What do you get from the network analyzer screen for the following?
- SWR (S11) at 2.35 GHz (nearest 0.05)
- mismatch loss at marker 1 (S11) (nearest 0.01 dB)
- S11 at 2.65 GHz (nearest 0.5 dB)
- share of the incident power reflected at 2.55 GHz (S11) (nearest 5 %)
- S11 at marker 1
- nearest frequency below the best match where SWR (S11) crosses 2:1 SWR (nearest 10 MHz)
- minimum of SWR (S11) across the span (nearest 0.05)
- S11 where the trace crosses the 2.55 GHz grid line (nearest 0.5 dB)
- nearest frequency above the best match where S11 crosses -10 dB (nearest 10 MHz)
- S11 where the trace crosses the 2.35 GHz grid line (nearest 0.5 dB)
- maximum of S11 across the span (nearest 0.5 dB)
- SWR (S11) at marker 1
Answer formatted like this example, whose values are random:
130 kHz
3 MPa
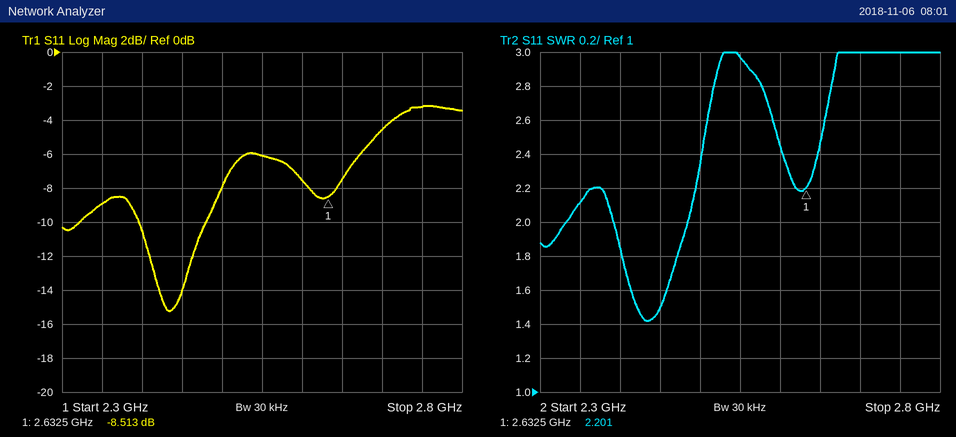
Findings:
2.10
0.66 dB
-7.5 dB
25 %
-8.513 dB
2.39 GHz
1.40
-6.0 dB
2.48 GHz
-9.0 dB
-3.0 dB
2.201
